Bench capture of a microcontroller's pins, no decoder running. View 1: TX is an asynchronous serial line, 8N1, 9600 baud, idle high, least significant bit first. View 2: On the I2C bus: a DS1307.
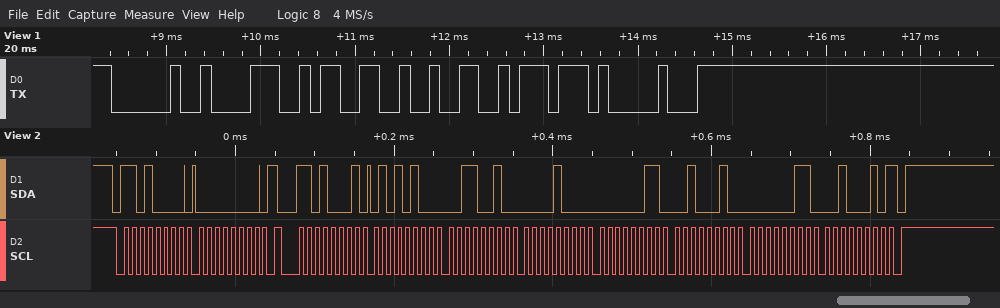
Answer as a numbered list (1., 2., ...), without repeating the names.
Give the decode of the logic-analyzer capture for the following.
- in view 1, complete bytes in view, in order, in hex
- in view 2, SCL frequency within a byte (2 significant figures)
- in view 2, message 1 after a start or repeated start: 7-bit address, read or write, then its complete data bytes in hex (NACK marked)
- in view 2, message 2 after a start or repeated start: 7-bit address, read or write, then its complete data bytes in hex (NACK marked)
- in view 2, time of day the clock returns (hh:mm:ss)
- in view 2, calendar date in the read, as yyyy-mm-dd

1. 20 38 33 32 77 10
2. 100 kHz
3. 0x68 write: 00
4. 0x68 read: 54 32 08 03 22 03 22 NACK
5. 08:32:54
6. 2022-03-22
